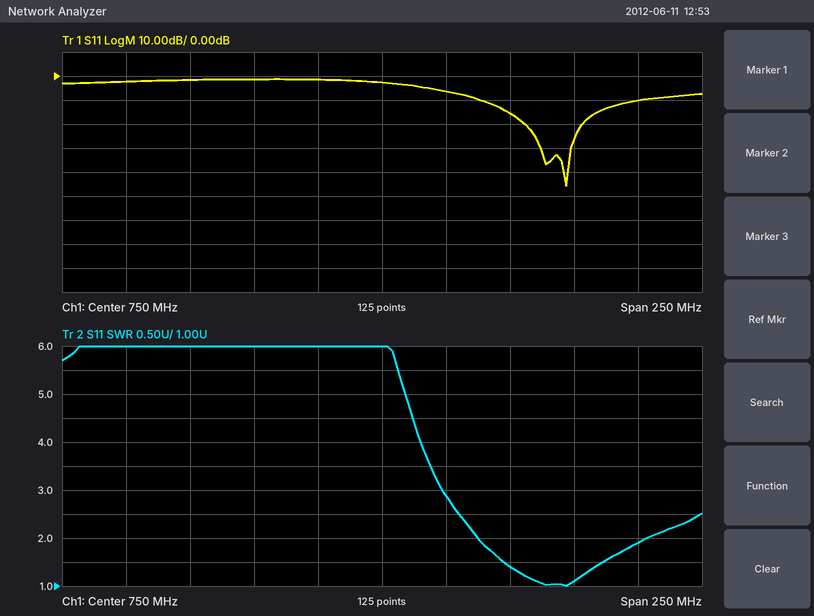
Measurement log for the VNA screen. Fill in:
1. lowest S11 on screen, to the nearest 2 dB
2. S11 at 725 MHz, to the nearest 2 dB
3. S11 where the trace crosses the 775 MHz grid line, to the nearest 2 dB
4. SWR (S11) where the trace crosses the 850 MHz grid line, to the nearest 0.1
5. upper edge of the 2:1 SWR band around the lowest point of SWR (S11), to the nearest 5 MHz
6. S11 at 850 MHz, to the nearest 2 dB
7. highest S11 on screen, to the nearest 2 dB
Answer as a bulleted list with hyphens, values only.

- -46 dB
- -2 dB
- -6 dB
- 1.9
- 855 MHz
- -10 dB
- -2 dB
